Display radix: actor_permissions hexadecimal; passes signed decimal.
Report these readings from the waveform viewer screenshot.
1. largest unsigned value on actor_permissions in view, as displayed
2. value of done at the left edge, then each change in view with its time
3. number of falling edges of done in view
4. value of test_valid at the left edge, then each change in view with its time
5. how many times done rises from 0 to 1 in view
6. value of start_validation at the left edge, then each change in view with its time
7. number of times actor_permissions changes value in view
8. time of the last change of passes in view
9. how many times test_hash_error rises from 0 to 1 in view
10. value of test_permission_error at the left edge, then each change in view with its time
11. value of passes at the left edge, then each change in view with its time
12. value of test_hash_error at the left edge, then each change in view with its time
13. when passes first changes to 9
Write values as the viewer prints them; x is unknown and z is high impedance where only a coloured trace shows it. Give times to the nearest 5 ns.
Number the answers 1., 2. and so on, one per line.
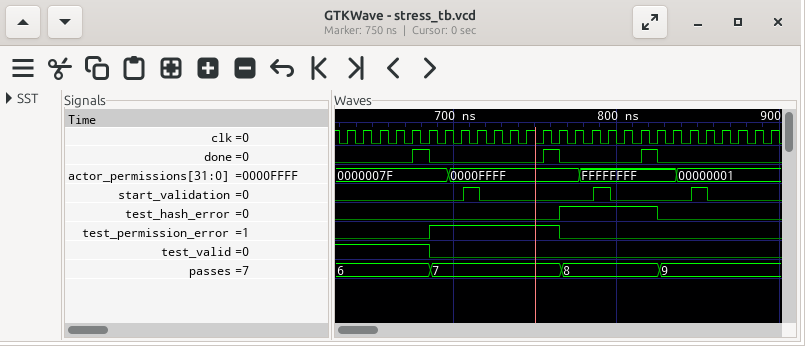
1. FFFFFFFF
2. 0, 1 at 675 ns, 0 at 685 ns, 1 at 755 ns, 0 at 765 ns, 1 at 815 ns, 0 at 825 ns
3. 3
4. 1, 0 at 685 ns
5. 3
6. 0, 1 at 705 ns, 0 at 715 ns, 1 at 785 ns, 0 at 795 ns, 1 at 845 ns, 0 at 855 ns
7. 3
8. 825 ns
9. 1
10. 0, 1 at 685 ns, 0 at 765 ns
11. 6, 7 at 685 ns, 8 at 765 ns, 9 at 825 ns
12. 0, 1 at 765 ns, 0 at 825 ns
13. 825 ns
